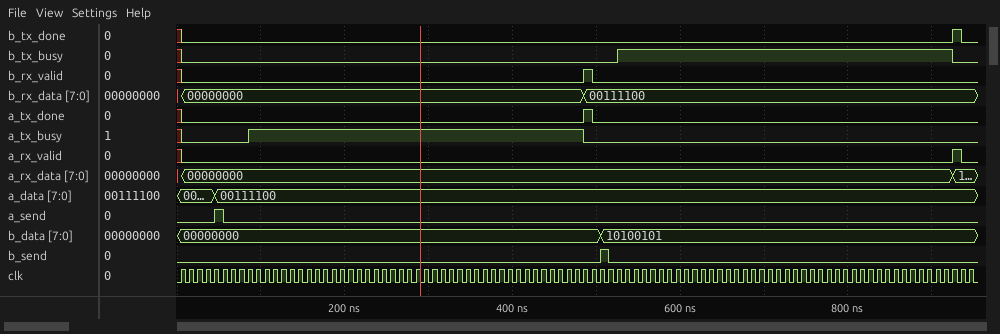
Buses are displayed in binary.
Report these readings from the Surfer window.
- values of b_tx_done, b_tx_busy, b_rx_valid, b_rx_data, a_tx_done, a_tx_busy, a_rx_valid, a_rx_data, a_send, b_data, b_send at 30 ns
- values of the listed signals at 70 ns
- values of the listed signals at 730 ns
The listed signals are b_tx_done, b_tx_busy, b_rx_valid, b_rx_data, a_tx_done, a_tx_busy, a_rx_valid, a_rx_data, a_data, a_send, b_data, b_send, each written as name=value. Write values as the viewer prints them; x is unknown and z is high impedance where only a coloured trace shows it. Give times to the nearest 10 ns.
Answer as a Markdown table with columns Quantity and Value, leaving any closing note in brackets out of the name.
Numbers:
| Quantity | Value |
|---|---|
| values of b_tx_done, b_tx_busy, b_rx_valid, b_rx_data, a_tx_done, a_tx_busy, a_rx_valid, a_rx_data, a_send, b_data, b_send at 30 ns | b_tx_done=0, b_tx_busy=0, b_rx_valid=0, b_rx_data=00000000, a_tx_done=0, a_tx_busy=0, a_rx_valid=0, a_rx_data=00000000, a_send=0, b_data=00000000, b_send=0 |
| values of the listed signals at 70 ns | b_tx_done=0, b_tx_busy=0, b_rx_valid=0, b_rx_data=00000000, a_tx_done=0, a_tx_busy=0, a_rx_valid=0, a_rx_data=00000000, a_data=00111100, a_send=0, b_data=00000000, b_send=0 |
| values of the listed signals at 730 ns | b_tx_done=0, b_tx_busy=1, b_rx_valid=0, b_rx_data=00111100, a_tx_done=0, a_tx_busy=0, a_rx_valid=0, a_rx_data=00000000, a_data=00111100, a_send=0, b_data=10100101, b_send=0 |
